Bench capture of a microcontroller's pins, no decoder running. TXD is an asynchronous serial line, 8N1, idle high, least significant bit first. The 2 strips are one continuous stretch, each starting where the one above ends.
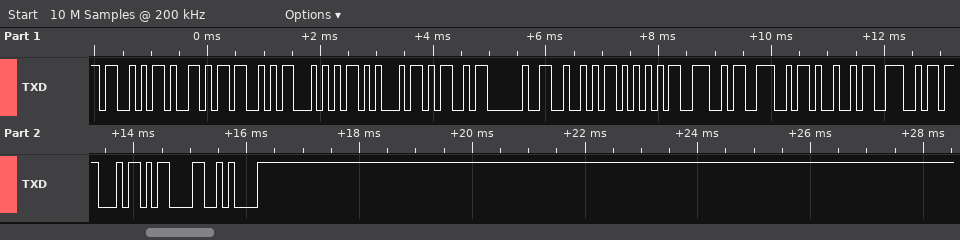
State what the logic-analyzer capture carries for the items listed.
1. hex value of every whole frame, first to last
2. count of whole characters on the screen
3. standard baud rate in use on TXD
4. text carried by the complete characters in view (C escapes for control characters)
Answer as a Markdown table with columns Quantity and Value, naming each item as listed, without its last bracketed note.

| Quantity | Value |
|---|---|
| hex value of every whole frame, first to last | 53 59 53 54 45 4D 20 52 55 4E 4E 49 4E 47 0D 0A |
| count of whole characters on the screen | 16 |
| standard baud rate in use on TXD | 9600 baud |
| text carried by the complete characters in view | "SYSTEM RUNNING\r\n" |
